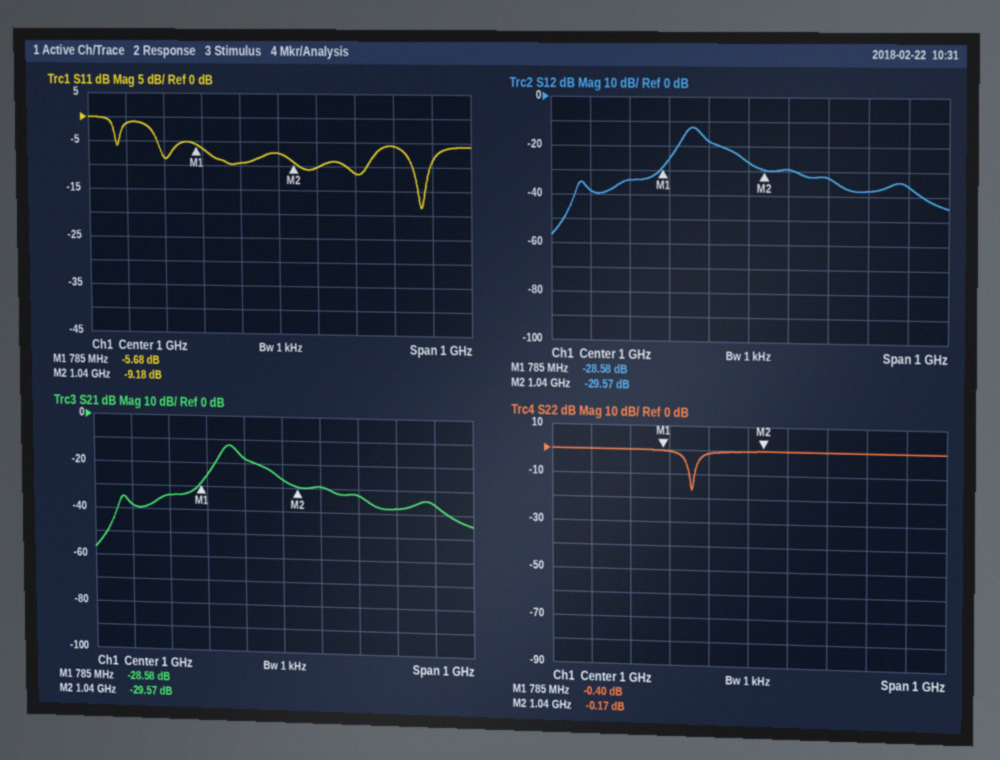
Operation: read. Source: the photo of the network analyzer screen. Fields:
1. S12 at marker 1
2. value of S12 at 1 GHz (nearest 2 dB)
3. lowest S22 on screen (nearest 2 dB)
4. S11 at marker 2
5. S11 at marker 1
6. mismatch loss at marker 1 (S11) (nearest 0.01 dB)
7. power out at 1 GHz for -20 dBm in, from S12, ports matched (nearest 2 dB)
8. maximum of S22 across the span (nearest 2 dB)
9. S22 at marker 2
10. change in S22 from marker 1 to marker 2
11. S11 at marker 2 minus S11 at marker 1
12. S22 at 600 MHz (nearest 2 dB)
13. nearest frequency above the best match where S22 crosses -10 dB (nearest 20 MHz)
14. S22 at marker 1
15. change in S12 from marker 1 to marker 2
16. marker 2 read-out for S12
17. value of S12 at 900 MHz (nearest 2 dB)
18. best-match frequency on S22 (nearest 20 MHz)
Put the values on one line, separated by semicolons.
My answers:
-28.58 dB; -26 dB; -16 dB; -9.18 dB; -5.68 dB; 1.37 dB; -46 dBm; 0 dB; -0.17 dB; 0.23 dB; -3.50 dB; 0 dB; 860 MHz; -0.40 dB; -0.99 dB; -29.57 dB; -18 dB; 860 MHz
